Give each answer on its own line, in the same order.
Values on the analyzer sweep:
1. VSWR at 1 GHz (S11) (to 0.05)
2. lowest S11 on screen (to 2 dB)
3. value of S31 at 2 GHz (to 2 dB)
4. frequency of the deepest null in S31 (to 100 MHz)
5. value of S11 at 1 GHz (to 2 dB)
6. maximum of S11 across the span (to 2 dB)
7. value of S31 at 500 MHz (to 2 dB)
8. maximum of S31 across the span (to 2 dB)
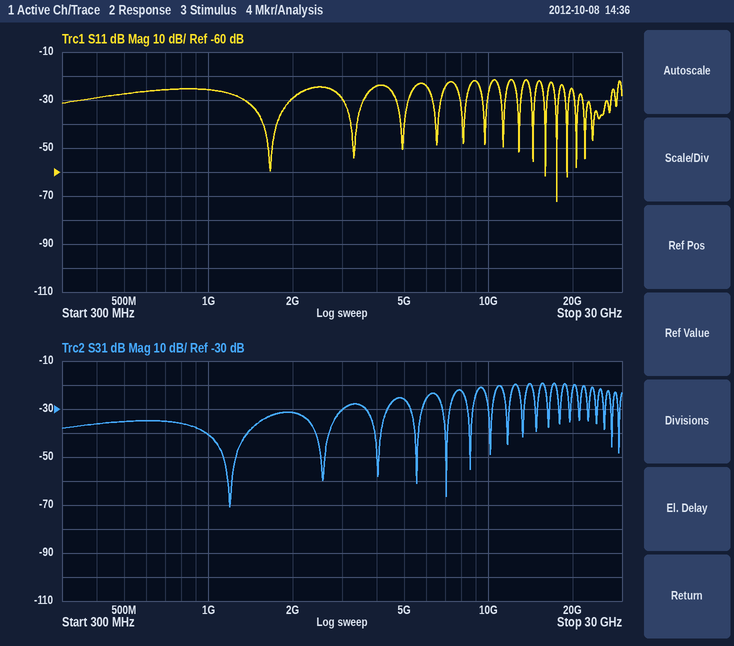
1.10
-72 dB
-32 dB
1.2 GHz
-26 dB
-22 dB
-36 dB
-20 dB
